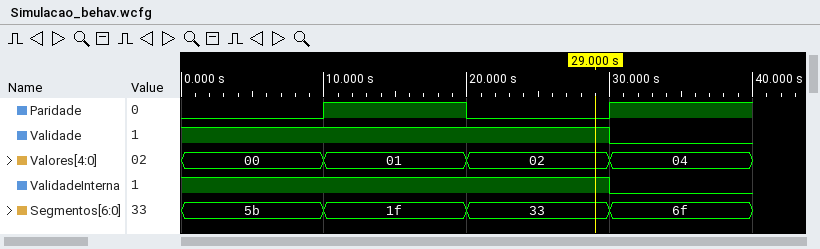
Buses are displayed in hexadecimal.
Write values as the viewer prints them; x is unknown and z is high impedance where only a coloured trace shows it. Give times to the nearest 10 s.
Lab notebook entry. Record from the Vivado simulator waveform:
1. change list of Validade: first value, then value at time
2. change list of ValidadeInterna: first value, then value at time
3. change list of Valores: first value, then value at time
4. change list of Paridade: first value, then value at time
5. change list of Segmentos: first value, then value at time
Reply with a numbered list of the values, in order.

1. 1, 0 at 30 s
2. 1, 0 at 30 s
3. 00, 01 at 10 s, 02 at 20 s, 04 at 30 s
4. 0, 1 at 10 s, 0 at 20 s, 1 at 30 s
5. 5b, 1f at 10 s, 33 at 20 s, 6f at 30 s
